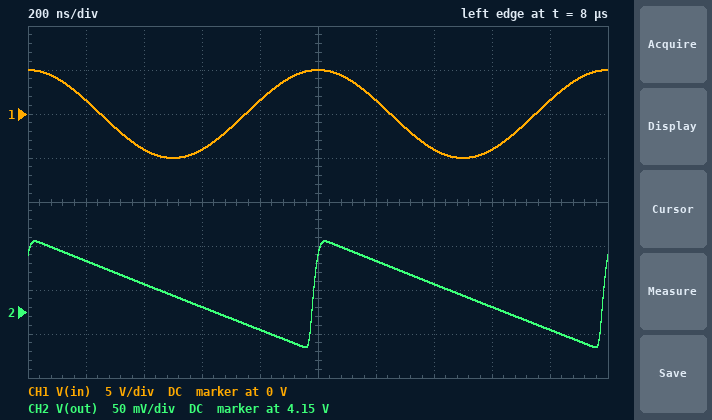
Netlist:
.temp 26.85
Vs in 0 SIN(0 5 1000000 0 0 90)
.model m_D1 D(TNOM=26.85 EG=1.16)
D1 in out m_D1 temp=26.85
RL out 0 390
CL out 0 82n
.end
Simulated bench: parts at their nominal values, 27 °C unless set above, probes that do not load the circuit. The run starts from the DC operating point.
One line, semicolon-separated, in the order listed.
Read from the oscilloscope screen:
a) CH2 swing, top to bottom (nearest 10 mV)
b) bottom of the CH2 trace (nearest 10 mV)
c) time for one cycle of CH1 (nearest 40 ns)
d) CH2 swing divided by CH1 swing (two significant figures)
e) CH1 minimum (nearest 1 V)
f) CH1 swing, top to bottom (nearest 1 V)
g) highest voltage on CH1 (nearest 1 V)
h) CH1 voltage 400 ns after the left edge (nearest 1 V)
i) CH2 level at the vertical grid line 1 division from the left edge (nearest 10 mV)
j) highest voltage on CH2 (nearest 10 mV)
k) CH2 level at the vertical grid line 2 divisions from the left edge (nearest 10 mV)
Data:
120 mV; 4.11 V; 1.00 µs; 0.012; -5 V; 10 V; 5 V; -4 V; 4.21 V; 4.23 V; 4.18 V
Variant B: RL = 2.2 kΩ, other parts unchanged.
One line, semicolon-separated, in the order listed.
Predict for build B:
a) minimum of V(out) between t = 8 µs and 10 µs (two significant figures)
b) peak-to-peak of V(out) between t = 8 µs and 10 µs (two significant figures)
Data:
4.2 V; 22 mV
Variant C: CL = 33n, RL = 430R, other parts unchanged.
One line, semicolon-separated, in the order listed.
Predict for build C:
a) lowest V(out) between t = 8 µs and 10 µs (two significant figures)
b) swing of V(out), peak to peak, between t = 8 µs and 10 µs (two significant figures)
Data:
4.0 V; 270 mV
